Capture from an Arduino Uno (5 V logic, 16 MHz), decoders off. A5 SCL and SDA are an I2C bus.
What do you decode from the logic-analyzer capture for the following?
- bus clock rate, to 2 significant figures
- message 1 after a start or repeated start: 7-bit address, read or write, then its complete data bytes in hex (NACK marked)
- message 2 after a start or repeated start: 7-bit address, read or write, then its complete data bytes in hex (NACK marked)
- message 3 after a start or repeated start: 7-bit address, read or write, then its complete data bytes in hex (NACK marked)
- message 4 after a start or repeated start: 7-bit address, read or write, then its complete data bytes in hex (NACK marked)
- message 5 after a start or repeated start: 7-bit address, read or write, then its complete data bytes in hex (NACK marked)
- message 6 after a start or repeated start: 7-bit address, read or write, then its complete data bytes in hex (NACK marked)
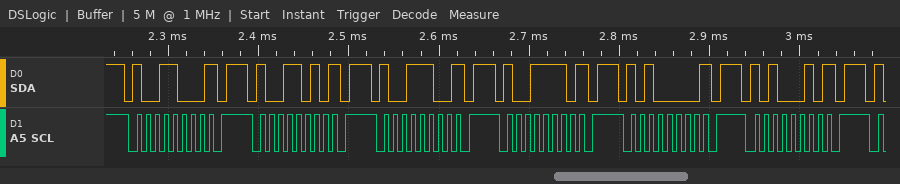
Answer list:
100 kHz
0x4C write NACK
0x4D write NACK
0x4E write NACK
0x4F write NACK
0x50 write NACK
0x51 write NACK
